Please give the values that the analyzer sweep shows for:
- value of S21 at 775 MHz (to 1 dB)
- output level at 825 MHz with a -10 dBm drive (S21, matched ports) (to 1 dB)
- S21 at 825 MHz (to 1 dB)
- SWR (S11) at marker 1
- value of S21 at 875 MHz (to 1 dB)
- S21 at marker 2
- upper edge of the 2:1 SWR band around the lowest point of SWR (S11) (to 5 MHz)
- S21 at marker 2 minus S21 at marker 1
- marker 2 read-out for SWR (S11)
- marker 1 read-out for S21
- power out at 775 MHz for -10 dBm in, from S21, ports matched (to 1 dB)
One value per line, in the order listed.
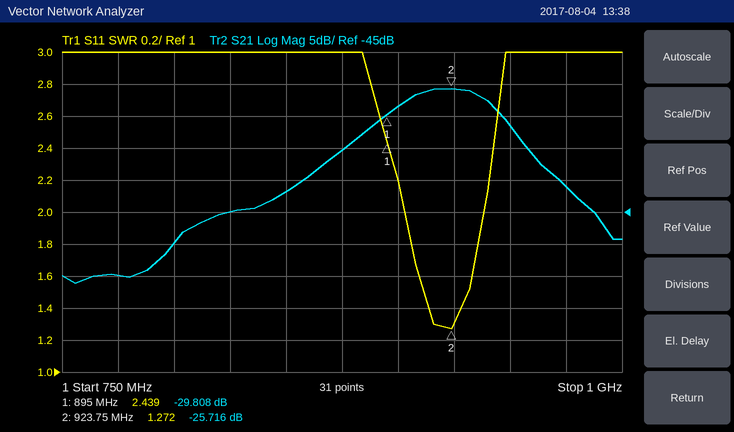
-55 dB
-55 dBm
-45 dB
2.439
-35 dB
-25.716 dB
940 MHz
4.092 dB
1.272
-29.808 dB
-65 dBm
